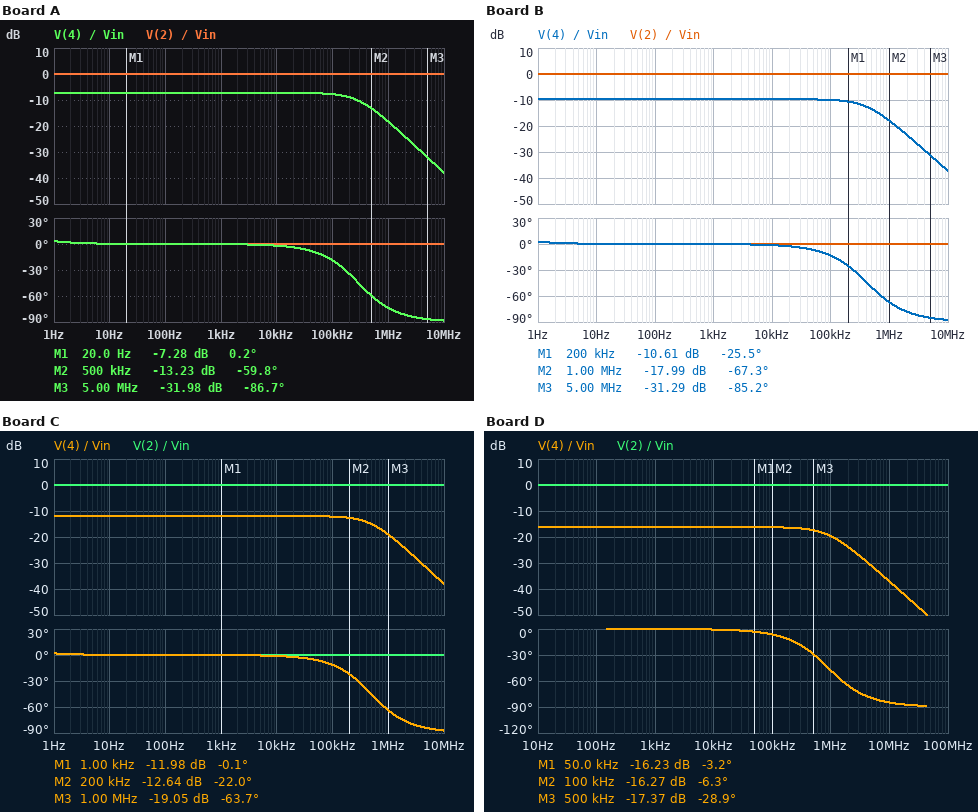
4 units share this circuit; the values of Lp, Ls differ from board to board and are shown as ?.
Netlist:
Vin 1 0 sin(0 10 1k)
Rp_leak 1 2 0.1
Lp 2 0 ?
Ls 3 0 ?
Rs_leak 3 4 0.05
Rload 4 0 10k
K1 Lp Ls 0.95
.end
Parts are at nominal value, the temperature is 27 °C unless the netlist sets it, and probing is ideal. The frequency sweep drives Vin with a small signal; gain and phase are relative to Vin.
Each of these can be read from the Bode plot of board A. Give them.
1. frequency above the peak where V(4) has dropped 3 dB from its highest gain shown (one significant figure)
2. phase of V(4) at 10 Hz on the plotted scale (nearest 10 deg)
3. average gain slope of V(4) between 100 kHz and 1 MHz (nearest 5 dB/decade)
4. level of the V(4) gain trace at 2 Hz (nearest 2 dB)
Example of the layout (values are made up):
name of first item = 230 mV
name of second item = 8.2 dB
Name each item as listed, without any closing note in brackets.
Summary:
frequency above the peak where V(4) has dropped 3 dB from its highest gain shown = 300 kHz
phase of V(4) at 10 Hz on the plotted scale = 0 deg
average gain slope of V(4) between 100 kHz and 1 MHz = -10 dB/decade
level of the V(4) gain trace at 2 Hz = -8 dB
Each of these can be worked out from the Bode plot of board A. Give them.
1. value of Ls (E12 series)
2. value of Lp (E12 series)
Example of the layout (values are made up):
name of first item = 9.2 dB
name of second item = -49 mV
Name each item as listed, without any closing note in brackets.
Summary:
value of Ls = 56 mH
value of Lp = 270 mH
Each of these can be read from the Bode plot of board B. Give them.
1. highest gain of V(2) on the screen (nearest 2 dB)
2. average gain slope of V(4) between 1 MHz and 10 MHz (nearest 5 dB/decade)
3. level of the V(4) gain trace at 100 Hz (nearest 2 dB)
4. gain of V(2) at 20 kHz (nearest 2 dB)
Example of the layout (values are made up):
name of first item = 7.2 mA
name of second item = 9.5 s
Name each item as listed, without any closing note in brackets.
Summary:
highest gain of V(2) on the screen = 0 dB
average gain slope of V(4) between 1 MHz and 10 MHz = -20 dB/decade
level of the V(4) gain trace at 100 Hz = -10 dB
gain of V(2) at 20 kHz = 0 dB
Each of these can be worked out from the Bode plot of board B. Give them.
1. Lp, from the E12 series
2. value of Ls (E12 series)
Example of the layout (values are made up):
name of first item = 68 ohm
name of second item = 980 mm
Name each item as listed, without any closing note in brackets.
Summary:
Lp, from the E12 series = 330 mH
value of Ls = 39 mH
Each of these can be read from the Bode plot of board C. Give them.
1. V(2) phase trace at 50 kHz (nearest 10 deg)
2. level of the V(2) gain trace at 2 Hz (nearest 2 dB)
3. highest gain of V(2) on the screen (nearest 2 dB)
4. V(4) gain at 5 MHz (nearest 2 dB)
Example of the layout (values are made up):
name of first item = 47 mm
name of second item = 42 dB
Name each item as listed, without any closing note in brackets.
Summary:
V(2) phase trace at 50 kHz = 0 deg
level of the V(2) gain trace at 2 Hz = 0 dB
highest gain of V(2) on the screen = 0 dB
V(4) gain at 5 MHz = -32 dB
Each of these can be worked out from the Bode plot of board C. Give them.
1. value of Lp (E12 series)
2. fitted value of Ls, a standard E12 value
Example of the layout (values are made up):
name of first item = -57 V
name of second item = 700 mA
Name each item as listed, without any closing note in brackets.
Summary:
value of Lp = 470 mH
fitted value of Ls, a standard E12 value = 33 mH
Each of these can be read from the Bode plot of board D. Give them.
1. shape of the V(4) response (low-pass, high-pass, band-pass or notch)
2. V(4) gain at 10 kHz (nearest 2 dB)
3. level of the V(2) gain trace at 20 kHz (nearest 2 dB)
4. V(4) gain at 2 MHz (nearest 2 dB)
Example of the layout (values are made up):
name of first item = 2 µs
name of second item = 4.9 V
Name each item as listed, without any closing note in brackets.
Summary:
shape of the V(4) response = low-pass
V(4) gain at 10 kHz = -16 dB
level of the V(2) gain trace at 20 kHz = 0 dB
V(4) gain at 2 MHz = -24 dB
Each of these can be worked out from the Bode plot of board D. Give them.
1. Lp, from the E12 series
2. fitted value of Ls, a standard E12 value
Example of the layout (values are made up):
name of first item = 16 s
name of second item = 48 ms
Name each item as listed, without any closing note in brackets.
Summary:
Lp, from the E12 series = 680 mH
fitted value of Ls, a standard E12 value = 18 mH
